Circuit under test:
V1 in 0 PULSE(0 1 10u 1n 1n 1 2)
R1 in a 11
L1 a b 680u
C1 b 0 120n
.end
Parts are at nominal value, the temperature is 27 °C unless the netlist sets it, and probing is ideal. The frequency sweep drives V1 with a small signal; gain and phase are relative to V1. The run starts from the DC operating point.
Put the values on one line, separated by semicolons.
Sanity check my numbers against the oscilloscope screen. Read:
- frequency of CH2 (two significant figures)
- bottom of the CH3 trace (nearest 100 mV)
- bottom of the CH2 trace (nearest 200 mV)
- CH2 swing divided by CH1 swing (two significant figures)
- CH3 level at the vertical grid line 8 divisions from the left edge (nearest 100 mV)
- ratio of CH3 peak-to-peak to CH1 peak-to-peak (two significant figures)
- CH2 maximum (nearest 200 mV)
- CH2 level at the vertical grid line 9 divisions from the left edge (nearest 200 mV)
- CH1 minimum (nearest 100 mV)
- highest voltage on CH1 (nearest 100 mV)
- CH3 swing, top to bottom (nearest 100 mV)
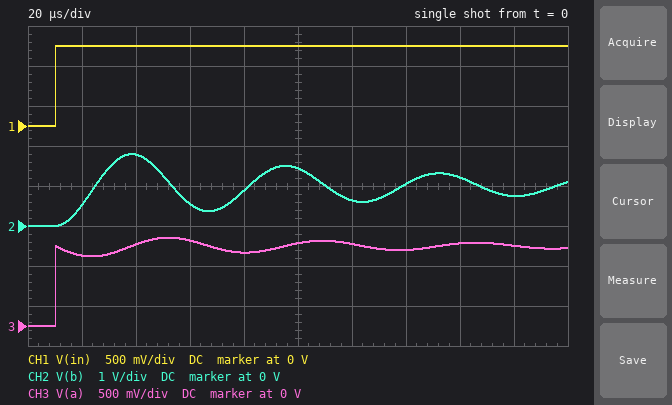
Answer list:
18 kHz; 0 V; 0 V; 1.8; 1.0 V; 1.1; 1.8 V; 800 mV; 0 V; 1.0 V; 1.1 V
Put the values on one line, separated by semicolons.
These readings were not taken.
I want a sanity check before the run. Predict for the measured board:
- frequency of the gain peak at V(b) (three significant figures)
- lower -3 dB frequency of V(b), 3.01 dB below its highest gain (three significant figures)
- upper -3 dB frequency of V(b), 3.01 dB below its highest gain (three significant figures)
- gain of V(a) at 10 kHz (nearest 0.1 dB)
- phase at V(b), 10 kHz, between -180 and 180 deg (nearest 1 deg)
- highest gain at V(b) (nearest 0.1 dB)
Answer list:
17.5 kHz; 16.2 kHz; 18.8 kHz; -0.1 dB; -7 deg; 16.7 dB
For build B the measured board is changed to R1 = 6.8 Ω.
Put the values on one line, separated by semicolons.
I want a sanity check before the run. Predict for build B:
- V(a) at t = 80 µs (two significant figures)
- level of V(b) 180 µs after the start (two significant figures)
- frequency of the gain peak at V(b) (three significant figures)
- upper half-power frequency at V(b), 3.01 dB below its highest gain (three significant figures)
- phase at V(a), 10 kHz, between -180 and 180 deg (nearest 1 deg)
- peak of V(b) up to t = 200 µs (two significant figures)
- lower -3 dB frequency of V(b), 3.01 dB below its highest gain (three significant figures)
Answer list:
940 mV; 570 mV; 17.6 kHz; 18.4 kHz; -4 deg; 1.9 V; 16.8 kHz
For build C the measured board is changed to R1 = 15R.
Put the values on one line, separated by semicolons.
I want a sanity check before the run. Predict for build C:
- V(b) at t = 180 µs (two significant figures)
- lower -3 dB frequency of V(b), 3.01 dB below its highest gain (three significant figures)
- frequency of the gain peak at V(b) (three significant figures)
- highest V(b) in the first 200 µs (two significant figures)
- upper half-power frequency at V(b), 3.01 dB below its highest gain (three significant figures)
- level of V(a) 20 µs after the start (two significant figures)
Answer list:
850 mV; 15.6 kHz; 17.4 kHz; 1.7 V; 19.1 kHz; 840 mV
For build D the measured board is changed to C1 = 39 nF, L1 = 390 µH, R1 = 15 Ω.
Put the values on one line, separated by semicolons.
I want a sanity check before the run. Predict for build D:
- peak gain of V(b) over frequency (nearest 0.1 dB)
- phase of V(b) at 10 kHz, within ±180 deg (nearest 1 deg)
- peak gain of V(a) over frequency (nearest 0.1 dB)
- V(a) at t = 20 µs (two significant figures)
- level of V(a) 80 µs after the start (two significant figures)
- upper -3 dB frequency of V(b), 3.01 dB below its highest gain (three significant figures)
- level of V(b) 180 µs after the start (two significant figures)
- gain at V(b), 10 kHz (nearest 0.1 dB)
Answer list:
16.5 dB; -2 deg; 0 dB; 930 mV; 1.0 V; 43.5 kHz; 970 mV; 0.5 dB
